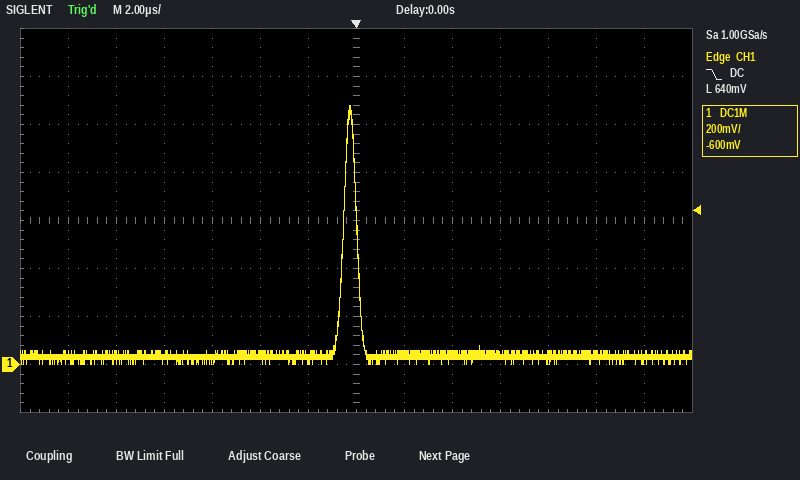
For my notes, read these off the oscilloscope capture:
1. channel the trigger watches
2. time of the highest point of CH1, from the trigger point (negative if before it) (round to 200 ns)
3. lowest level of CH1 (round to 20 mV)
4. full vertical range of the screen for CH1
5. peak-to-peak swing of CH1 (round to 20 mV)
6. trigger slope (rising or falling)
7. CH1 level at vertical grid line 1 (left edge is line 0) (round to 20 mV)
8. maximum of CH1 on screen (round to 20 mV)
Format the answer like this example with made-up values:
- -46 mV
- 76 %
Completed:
- CH1
- -200 ns
- 0 mV
- 1.6 V
- 1.08 V
- falling
- 40 mV
- 1.08 V
